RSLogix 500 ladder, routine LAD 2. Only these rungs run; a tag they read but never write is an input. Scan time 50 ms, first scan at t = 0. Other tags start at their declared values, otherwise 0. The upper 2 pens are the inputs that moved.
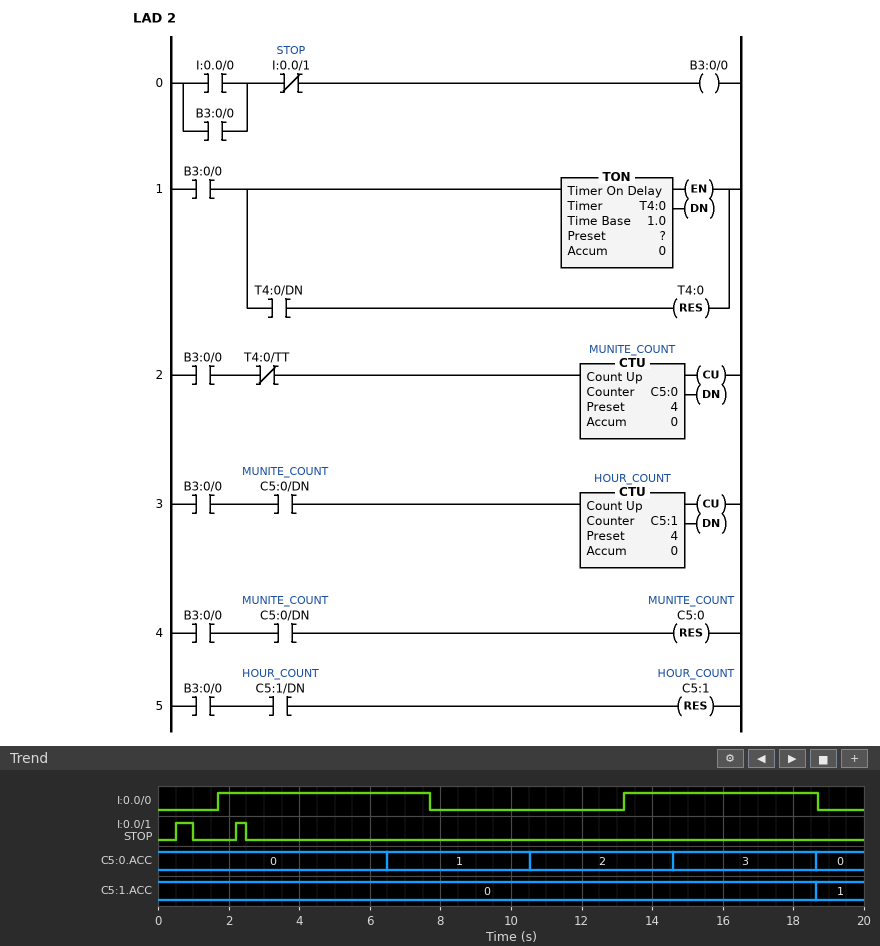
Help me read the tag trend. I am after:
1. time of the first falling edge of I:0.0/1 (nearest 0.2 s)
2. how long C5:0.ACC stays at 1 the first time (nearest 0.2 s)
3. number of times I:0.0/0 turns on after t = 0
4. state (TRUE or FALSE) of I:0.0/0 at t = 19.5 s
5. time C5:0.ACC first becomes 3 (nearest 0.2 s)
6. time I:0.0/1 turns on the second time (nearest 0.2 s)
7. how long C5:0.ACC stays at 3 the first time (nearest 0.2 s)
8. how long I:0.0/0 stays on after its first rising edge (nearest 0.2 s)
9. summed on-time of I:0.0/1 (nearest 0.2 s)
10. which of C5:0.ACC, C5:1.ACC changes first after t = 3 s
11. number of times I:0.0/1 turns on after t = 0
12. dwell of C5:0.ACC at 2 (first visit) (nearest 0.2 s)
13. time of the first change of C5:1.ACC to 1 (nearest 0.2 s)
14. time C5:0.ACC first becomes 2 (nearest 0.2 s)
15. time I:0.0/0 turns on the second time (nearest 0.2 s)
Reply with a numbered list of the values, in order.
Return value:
1. 1.0 s
2. 4.0 s
3. 2
4. FALSE
5. 14.6 s
6. 2.2 s
7. 4.0 s
8. 6.0 s
9. 0.8 s
10. C5:0.ACC
11. 2
12. 4.0 s
13. 18.6 s
14. 10.6 s
15. 13.2 s
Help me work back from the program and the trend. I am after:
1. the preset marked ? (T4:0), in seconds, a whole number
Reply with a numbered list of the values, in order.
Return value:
1. 4 s
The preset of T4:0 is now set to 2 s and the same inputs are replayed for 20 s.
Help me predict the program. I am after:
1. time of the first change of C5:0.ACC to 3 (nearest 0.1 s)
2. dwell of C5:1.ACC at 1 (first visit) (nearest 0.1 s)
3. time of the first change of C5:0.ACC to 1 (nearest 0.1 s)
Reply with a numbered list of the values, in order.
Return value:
1. 8.6 s
2. 8.2 s
3. 4.5 s
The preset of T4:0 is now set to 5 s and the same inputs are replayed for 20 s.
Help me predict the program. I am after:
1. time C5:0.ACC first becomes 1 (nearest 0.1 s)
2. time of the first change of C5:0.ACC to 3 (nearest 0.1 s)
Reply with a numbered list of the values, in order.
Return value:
1. 7.5 s
2. 17.6 s
